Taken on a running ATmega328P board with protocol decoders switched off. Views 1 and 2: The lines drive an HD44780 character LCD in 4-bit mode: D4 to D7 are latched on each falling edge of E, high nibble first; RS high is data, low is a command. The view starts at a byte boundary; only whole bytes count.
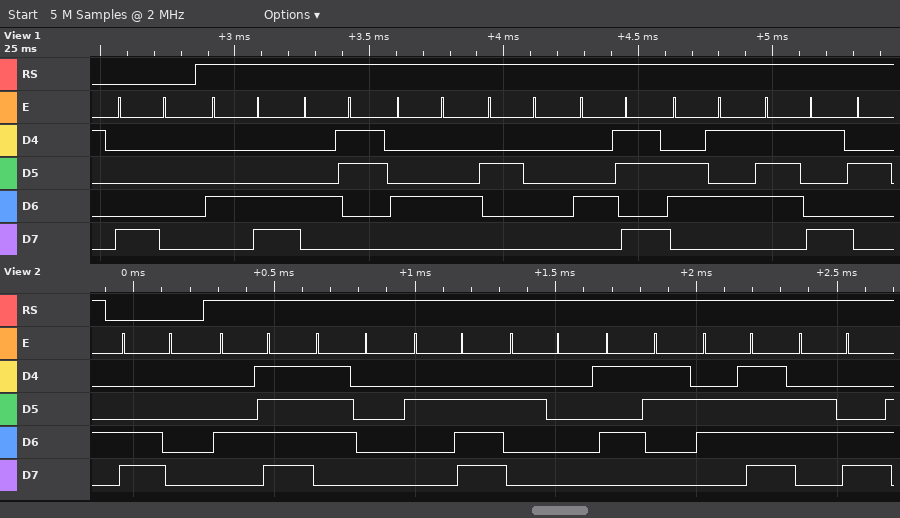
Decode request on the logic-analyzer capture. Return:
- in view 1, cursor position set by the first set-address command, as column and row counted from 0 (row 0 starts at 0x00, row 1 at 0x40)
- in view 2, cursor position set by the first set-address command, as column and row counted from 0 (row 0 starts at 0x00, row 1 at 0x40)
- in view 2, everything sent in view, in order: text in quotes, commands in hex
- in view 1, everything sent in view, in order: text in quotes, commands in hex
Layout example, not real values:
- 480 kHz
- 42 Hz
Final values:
- column 0, row 0
- column 0, row 1
- 0xC0 "Op. Sol"
- 0x80 "LCD Key"
